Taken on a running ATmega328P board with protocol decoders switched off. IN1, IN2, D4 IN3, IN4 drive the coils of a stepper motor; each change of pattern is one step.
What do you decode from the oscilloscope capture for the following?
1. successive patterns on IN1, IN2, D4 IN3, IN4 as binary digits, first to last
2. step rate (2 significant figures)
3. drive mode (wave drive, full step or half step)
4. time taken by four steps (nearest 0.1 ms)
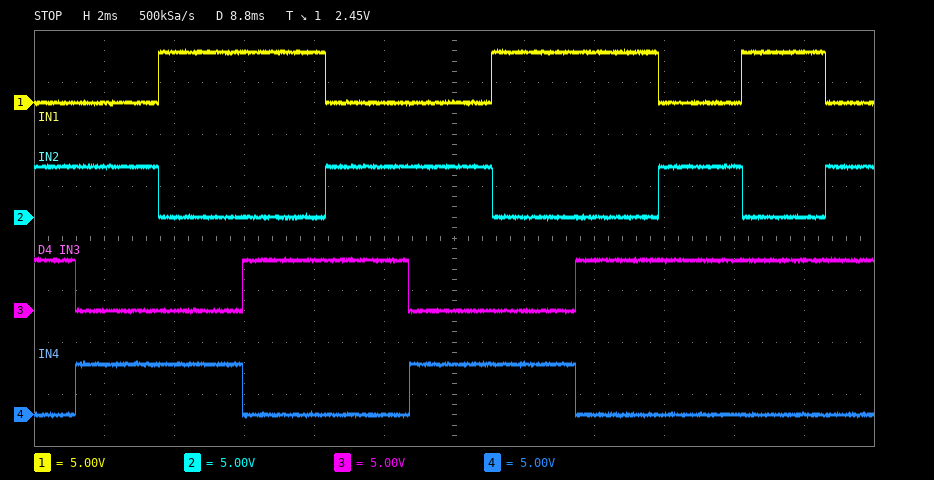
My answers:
0110 0101 1001 1010 0110 0101 1001 1010 0110 1010 0110
420 steps/s
full step
9.5 ms
